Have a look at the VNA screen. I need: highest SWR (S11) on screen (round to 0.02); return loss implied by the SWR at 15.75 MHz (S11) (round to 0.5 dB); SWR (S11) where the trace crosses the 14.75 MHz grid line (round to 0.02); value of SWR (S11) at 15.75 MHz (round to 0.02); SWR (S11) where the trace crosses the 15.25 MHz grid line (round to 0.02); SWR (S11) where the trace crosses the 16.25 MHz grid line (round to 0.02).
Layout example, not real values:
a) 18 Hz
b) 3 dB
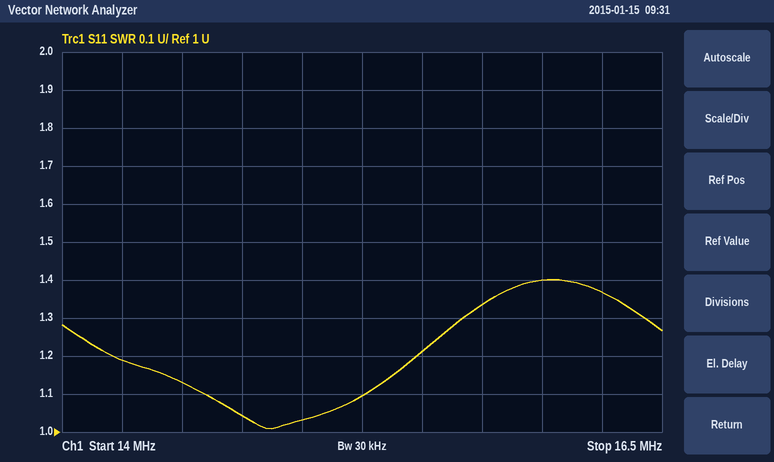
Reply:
a) 1.40
b) 17.0 dB
c) 1.04
d) 1.34
e) 1.10
f) 1.36
